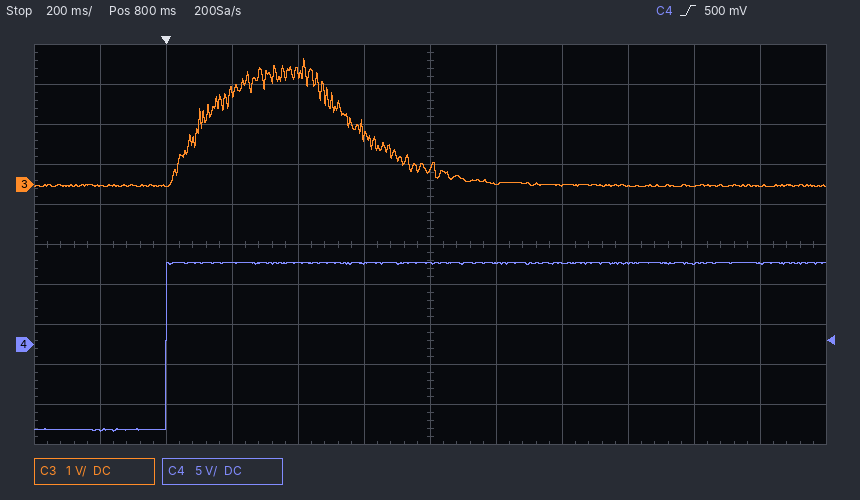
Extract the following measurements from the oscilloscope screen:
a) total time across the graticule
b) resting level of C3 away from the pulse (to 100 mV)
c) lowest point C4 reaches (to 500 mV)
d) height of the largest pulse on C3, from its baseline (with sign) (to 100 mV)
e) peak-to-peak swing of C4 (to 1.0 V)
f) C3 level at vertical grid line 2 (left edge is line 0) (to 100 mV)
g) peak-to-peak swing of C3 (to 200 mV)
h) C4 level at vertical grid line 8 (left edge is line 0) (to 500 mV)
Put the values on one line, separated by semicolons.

2.4 s; 0.0 V; -11.0 V; +3.2 V; 21.0 V; 0.0 V; 3.2 V; 10.0 V
